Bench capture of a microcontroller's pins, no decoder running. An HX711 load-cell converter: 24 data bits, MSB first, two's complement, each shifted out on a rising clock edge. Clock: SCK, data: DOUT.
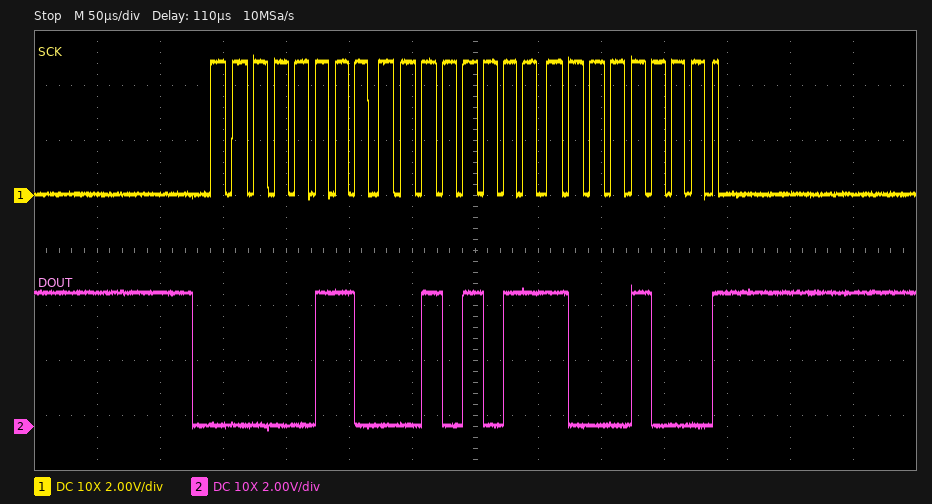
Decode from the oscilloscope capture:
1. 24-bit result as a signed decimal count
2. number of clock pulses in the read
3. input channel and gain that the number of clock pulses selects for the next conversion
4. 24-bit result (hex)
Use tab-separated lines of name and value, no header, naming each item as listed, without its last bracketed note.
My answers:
24-bit result as a signed decimal count	404360
number of clock pulses in the read	25
input channel and gain that the number of clock pulses selects for the next conversion	channel A, gain 128
24-bit result	0x062B88
